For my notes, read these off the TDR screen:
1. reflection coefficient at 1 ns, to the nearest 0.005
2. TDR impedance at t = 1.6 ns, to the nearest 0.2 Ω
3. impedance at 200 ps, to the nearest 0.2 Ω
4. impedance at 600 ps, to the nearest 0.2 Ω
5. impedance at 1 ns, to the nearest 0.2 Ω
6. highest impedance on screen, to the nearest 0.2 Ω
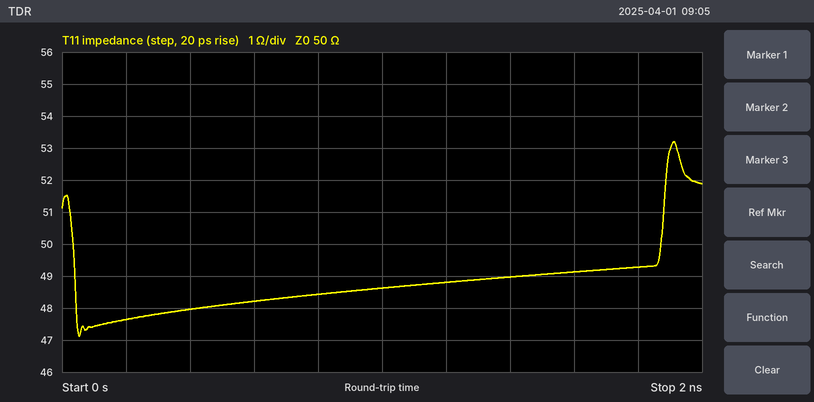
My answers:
-0.015
49.2 Ω
47.6 Ω
48.2 Ω
48.6 Ω
53.2 Ω
